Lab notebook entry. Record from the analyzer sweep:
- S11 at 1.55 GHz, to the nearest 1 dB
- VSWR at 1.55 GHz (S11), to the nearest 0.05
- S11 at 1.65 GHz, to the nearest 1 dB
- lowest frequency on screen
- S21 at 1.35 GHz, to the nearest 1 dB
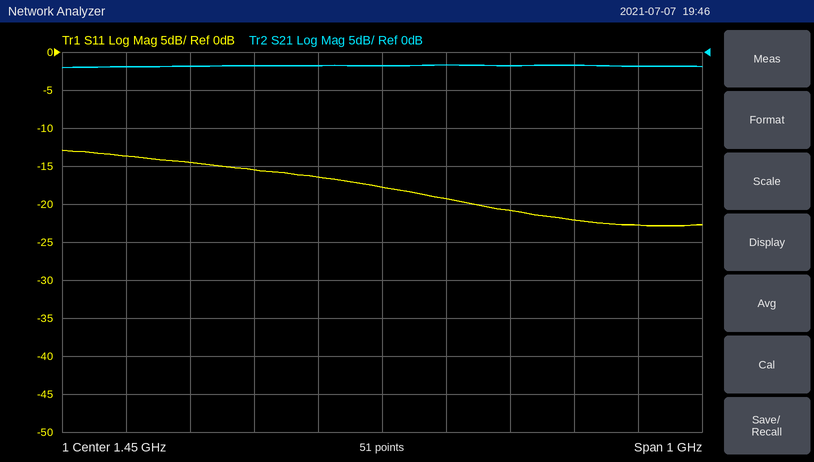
-19 dB
1.25
-21 dB
950 MHz
-2 dB
